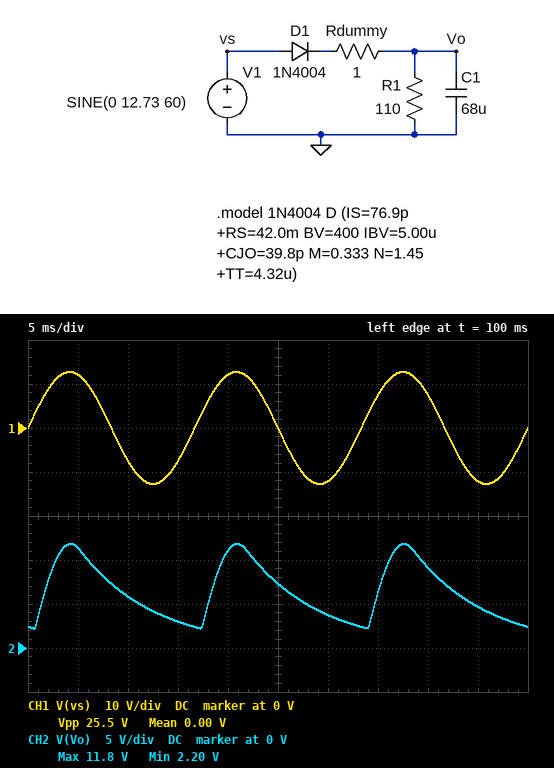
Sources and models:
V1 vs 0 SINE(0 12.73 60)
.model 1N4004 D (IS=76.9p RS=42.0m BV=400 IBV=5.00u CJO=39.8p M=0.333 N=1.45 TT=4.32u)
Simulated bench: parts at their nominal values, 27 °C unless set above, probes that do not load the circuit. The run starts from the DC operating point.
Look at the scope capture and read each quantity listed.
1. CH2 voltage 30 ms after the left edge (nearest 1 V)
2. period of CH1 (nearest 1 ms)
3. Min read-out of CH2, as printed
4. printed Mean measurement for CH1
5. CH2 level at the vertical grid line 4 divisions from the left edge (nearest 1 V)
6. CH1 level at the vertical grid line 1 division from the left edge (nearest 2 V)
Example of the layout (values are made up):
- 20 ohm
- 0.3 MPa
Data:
- 4 V
- 17 ms
- 2.20 V
- 0.00 V
- 11 V
- 12 V
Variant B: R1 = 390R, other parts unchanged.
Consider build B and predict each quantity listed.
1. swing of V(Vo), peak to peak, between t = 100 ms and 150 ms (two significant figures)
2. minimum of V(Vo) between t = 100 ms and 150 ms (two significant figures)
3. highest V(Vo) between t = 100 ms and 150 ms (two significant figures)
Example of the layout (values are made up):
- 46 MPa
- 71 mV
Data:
- 4.9 V
- 7.1 V
- 12 V
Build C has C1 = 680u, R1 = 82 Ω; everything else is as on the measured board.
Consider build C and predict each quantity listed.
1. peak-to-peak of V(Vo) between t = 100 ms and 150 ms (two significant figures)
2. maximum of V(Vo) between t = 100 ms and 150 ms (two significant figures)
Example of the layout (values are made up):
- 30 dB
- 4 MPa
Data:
- 2.5 V
- 11 V
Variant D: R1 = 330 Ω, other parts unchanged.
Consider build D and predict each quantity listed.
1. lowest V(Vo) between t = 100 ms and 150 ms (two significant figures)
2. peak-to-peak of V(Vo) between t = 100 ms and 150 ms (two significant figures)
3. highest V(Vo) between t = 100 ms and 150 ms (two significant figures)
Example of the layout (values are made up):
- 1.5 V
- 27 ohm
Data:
- 6.5 V
- 5.5 V
- 12 V
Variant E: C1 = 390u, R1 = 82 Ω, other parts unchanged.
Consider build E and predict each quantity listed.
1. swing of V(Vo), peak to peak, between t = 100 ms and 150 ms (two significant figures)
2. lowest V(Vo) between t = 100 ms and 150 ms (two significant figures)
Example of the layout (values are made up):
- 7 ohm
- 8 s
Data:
- 4.1 V
- 7.5 V
